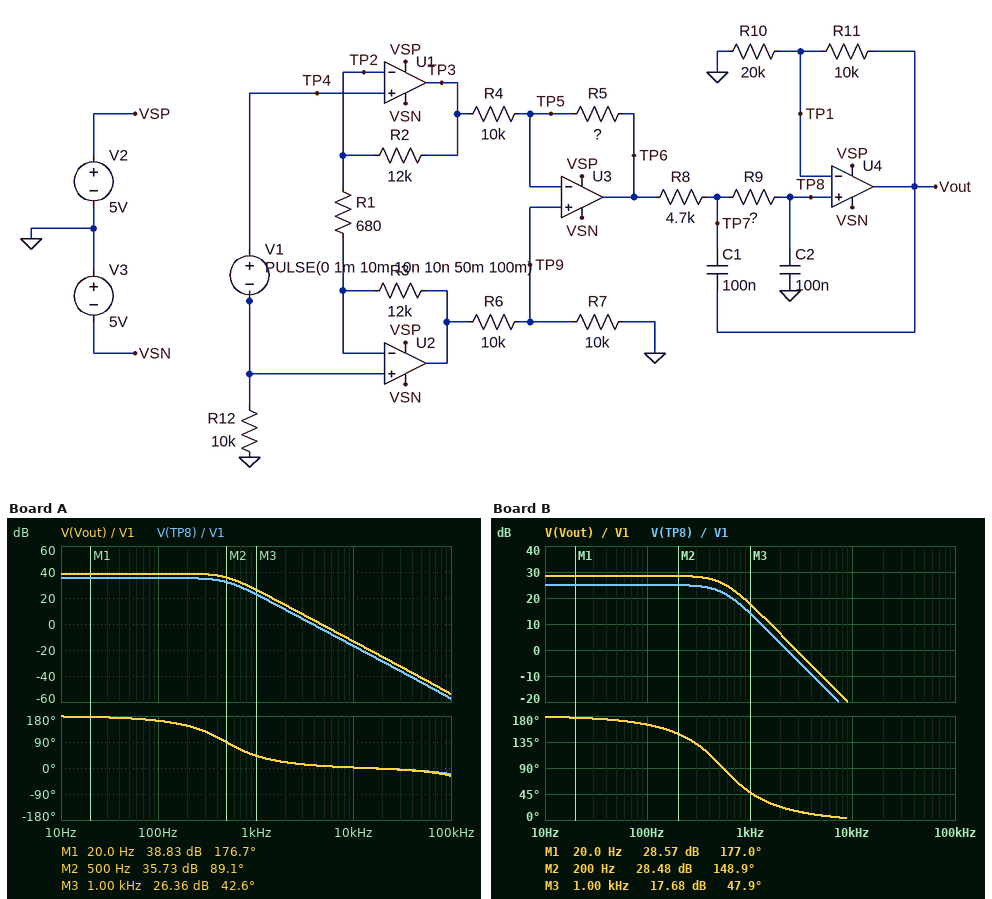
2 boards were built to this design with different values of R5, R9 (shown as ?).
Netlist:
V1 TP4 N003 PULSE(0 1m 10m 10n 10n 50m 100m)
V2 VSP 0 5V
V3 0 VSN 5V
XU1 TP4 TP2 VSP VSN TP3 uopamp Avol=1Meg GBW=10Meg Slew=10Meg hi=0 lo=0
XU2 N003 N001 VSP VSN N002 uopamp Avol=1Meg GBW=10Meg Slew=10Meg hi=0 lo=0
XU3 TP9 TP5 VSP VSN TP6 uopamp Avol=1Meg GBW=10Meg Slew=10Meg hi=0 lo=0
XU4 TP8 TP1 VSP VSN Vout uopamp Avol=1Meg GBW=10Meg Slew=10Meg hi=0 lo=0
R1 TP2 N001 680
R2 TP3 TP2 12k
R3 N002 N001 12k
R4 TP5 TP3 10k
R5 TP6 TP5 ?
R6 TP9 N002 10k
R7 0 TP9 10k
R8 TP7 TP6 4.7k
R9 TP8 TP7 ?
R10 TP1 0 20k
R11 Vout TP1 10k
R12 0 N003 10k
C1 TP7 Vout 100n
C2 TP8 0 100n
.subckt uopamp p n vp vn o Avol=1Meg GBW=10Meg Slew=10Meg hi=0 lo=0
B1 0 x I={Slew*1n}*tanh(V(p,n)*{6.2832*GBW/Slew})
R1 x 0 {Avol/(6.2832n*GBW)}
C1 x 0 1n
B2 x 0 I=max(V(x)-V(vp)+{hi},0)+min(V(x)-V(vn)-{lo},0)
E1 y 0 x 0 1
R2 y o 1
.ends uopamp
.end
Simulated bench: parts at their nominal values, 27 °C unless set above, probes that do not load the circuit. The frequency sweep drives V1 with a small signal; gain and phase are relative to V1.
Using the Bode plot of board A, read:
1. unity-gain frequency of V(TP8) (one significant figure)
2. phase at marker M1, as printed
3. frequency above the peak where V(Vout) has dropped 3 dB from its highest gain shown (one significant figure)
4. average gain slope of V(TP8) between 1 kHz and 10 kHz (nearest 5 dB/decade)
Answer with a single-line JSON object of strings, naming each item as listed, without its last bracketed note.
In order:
{"unity-gain frequency of V(TP8)": "4 kHz", "phase at marker M1, as printed": "176.7 deg", "frequency above the peak where V(Vout) has dropped 3 dB from its highest gain shown": "500 Hz", "average gain slope of V(TP8) between 1 kHz and 10 kHz": "-40 dB/decade"}
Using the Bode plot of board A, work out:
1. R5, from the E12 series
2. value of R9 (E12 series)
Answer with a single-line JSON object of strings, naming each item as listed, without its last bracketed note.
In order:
{"R5, from the E12 series": "18 kΩ", "value of R9": "2.2 kΩ"}
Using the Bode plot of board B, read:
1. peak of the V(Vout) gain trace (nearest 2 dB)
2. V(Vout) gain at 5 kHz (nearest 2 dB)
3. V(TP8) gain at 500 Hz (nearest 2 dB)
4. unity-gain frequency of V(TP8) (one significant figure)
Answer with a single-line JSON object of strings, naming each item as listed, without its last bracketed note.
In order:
{"peak of the V(Vout) gain trace": "28 dB", "V(Vout) gain at 5 kHz": "-10 dB", "V(TP8) gain at 500 Hz": "22 dB", "unity-gain frequency of V(TP8)": "2 kHz"}
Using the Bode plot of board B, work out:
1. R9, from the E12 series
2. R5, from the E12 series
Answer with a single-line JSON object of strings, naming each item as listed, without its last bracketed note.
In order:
{"R9, from the E12 series": "1.8 kΩ", "R5, from the E12 series": "3.3 kΩ"}
